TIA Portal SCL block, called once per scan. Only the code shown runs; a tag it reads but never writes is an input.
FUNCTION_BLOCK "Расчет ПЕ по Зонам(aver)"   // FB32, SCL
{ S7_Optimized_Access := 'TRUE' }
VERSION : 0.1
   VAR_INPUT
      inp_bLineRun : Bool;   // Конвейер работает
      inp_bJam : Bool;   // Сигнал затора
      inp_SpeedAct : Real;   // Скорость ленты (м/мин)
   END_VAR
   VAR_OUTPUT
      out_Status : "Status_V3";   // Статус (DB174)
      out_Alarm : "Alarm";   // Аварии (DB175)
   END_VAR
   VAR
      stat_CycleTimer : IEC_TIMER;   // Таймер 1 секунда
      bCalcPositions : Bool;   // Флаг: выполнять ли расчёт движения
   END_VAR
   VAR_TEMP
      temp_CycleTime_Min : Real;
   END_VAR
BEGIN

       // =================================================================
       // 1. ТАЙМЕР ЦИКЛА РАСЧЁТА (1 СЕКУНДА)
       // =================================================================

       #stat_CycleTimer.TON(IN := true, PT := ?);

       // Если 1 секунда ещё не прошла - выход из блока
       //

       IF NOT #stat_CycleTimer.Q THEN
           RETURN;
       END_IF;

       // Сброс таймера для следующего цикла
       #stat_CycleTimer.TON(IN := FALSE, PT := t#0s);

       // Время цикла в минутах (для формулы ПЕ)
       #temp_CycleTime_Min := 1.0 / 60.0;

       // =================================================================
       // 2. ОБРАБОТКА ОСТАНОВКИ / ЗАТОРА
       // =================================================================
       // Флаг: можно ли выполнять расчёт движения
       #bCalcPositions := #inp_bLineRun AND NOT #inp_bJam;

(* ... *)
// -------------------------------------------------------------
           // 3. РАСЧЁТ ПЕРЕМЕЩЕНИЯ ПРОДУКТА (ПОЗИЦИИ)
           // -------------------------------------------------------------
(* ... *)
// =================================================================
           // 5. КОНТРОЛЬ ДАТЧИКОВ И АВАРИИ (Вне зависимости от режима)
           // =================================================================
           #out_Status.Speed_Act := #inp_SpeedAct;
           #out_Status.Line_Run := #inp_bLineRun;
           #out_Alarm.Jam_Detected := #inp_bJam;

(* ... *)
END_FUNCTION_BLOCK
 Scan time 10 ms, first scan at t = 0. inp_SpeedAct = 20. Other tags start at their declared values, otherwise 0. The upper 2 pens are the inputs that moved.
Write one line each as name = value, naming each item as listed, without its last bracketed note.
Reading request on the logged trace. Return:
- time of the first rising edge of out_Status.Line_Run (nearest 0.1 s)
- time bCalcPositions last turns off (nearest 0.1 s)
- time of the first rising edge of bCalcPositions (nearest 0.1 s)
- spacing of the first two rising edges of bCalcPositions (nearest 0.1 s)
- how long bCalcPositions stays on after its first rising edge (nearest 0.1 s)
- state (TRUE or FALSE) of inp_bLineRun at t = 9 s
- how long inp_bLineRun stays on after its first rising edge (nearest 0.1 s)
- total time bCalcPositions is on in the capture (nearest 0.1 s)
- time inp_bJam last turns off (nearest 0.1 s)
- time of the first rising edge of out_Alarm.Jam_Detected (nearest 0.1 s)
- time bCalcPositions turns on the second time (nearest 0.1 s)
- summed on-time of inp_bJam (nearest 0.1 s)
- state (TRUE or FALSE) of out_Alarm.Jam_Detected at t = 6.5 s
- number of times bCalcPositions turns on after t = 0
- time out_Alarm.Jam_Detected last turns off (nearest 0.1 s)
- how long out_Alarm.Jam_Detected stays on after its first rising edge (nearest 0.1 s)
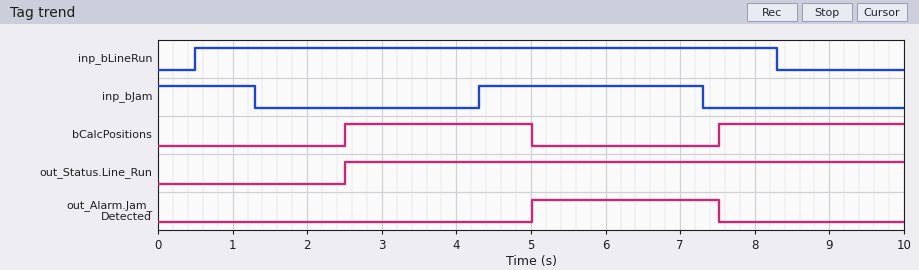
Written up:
time of the first rising edge of out_Status.Line_Run = 2.5 s
time bCalcPositions last turns off = 5.0 s
time of the first rising edge of bCalcPositions = 2.5 s
spacing of the first two rising edges of bCalcPositions = 5.0 s
how long bCalcPositions stays on after its first rising edge = 2.5 s
state (TRUE or FALSE) of inp_bLineRun at t = 9 s = FALSE
how long inp_bLineRun stays on after its first rising edge = 7.8 s
total time bCalcPositions is on in the capture = 5.0 s
time inp_bJam last turns off = 7.3 s
time of the first rising edge of out_Alarm.Jam_Detected = 5.0 s
time bCalcPositions turns on the second time = 7.5 s
summed on-time of inp_bJam = 4.3 s
state (TRUE or FALSE) of out_Alarm.Jam_Detected at t = 6.5 s = TRUE
number of times bCalcPositions turns on after t = 0 = 2
time out_Alarm.Jam_Detected last turns off = 7.5 s
how long out_Alarm.Jam_Detected stays on after its first rising edge = 2.5 s
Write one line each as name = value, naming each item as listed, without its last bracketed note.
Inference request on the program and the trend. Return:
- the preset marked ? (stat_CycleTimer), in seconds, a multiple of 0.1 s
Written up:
the preset marked ? (stat_CycleTimer), in seconds, a multiple of 0.1 s = 2.5 s
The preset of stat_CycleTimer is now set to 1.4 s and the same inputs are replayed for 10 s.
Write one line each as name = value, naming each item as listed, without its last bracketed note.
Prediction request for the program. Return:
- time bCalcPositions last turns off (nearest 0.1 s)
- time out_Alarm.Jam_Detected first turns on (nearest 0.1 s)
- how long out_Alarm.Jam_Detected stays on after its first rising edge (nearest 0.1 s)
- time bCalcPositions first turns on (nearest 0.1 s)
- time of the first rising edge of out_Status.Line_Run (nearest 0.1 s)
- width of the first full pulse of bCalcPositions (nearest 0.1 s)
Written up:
time bCalcPositions last turns off = 5.6 s
time out_Alarm.Jam_Detected first turns on = 5.6 s
how long out_Alarm.Jam_Detected stays on after its first rising edge = 2.8 s
time bCalcPositions first turns on = 1.4 s
time of the first rising edge of out_Status.Line_Run = 1.4 s
width of the first full pulse of bCalcPositions = 4.2 s
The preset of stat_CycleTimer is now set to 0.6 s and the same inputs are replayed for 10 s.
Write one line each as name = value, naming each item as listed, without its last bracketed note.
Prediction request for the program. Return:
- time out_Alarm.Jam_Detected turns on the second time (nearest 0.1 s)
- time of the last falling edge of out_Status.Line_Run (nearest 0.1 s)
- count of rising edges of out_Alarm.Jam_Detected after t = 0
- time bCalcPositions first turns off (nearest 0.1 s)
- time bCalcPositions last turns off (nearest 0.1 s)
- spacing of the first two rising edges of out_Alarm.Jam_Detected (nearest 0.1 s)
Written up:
time out_Alarm.Jam_Detected turns on the second time = 4.9 s
time of the last falling edge of out_Status.Line_Run = 8.5 s
count of rising edges of out_Alarm.Jam_Detected after t = 0 = 2
time bCalcPositions first turns off = 4.9 s
time bCalcPositions last turns off = 8.5 s
spacing of the first two rising edges of out_Alarm.Jam_Detected = 4.3 s
